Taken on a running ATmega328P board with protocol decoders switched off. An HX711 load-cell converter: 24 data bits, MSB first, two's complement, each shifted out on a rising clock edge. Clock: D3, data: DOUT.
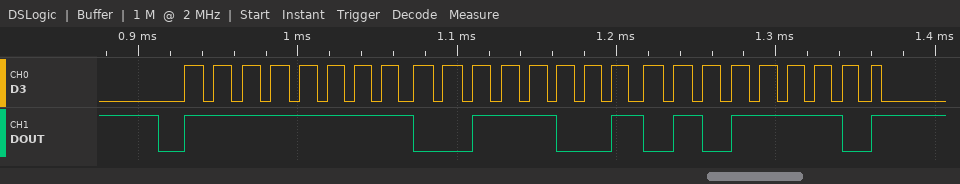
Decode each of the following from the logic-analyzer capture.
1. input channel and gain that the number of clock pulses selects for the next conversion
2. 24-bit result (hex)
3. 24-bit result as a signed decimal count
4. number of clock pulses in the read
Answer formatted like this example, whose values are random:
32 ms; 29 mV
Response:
channel A, gain 128; 0xFF395E; -50850; 25
